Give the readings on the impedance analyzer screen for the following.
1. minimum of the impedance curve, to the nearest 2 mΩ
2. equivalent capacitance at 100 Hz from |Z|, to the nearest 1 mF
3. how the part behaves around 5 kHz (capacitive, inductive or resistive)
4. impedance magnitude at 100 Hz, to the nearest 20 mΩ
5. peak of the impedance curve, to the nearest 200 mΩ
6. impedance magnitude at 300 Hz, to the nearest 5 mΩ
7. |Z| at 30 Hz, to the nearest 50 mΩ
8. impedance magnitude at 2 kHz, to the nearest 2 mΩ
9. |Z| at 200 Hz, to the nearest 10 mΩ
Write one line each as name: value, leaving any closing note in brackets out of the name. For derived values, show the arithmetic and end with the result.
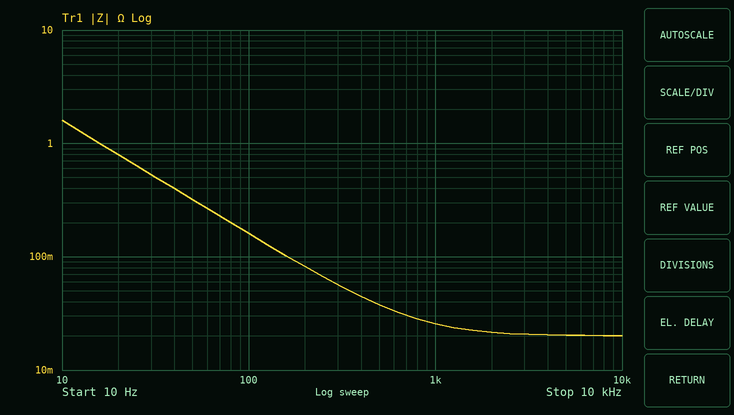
minimum of the impedance curve, to the nearest 2 mΩ: 20 mΩ
equivalent capacitance at 100 Hz from |Z|, to the nearest 1 mF: C = 1/(2π × 100 Hz × 160 mΩ) ≈ 10 mF
how the part behaves around 5 kHz: resistive
impedance magnitude at 100 Hz, to the nearest 20 mΩ: 160 mΩ
peak of the impedance curve, to the nearest 200 mΩ: 1.6 Ω
impedance magnitude at 300 Hz, to the nearest 5 mΩ: 55 mΩ
|Z| at 30 Hz, to the nearest 50 mΩ: 550 mΩ
impedance magnitude at 2 kHz, to the nearest 2 mΩ: 22 mΩ
|Z| at 200 Hz, to the nearest 10 mΩ: 80 mΩ
